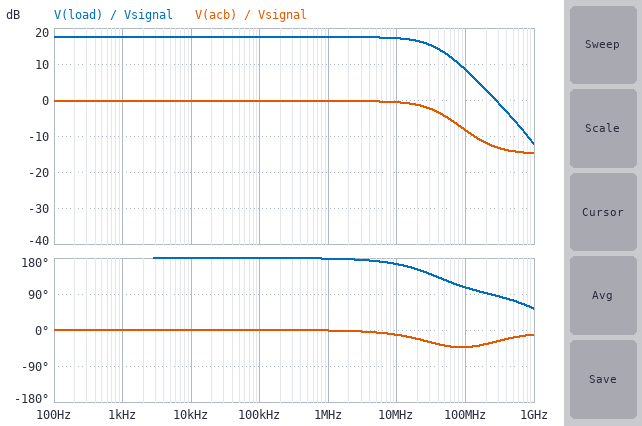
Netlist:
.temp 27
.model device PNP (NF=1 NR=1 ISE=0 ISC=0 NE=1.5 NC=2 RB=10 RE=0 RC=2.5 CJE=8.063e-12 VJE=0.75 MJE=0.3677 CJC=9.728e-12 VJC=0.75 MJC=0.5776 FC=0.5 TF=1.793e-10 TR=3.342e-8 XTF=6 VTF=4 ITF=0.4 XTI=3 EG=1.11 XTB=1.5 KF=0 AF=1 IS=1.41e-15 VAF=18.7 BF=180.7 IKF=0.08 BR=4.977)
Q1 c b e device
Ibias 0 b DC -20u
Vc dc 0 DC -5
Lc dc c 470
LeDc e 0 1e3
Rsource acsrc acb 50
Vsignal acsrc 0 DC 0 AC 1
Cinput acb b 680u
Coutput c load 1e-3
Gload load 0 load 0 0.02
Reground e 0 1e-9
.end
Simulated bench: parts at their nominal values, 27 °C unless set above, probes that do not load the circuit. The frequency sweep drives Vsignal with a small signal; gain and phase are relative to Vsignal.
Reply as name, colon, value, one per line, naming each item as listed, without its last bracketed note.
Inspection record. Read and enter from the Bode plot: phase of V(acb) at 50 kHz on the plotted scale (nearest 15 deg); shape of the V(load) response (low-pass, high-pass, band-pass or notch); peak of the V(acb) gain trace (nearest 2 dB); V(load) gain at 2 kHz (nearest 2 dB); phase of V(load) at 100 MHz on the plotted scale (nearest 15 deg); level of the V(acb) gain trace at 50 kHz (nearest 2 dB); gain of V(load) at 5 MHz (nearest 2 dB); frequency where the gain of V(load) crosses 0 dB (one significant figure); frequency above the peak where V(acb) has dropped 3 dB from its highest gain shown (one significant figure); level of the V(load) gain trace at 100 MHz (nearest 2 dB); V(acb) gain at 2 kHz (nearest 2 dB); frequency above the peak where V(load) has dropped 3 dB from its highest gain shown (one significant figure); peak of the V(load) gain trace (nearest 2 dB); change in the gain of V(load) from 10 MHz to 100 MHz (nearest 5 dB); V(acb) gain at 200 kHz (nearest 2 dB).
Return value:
phase of V(acb) at 50 kHz on the plotted scale: 0 deg
shape of the V(load) response: low-pass
peak of the V(acb) gain trace: 0 dB
V(load) gain at 2 kHz: 18 dB
phase of V(load) at 100 MHz on the plotted scale: 105 deg
level of the V(acb) gain trace at 50 kHz: 0 dB
gain of V(load) at 5 MHz: 18 dB
frequency where the gain of V(load) crosses 0 dB: 300 MHz
frequency above the peak where V(acb) has dropped 3 dB from its highest gain shown: 40 MHz
level of the V(load) gain trace at 100 MHz: 8 dB
V(acb) gain at 2 kHz: 0 dB
frequency above the peak where V(load) has dropped 3 dB from its highest gain shown: 40 MHz
peak of the V(load) gain trace: 18 dB
change in the gain of V(load) from 10 MHz to 100 MHz: -10 dB
V(acb) gain at 200 kHz: 0 dB
